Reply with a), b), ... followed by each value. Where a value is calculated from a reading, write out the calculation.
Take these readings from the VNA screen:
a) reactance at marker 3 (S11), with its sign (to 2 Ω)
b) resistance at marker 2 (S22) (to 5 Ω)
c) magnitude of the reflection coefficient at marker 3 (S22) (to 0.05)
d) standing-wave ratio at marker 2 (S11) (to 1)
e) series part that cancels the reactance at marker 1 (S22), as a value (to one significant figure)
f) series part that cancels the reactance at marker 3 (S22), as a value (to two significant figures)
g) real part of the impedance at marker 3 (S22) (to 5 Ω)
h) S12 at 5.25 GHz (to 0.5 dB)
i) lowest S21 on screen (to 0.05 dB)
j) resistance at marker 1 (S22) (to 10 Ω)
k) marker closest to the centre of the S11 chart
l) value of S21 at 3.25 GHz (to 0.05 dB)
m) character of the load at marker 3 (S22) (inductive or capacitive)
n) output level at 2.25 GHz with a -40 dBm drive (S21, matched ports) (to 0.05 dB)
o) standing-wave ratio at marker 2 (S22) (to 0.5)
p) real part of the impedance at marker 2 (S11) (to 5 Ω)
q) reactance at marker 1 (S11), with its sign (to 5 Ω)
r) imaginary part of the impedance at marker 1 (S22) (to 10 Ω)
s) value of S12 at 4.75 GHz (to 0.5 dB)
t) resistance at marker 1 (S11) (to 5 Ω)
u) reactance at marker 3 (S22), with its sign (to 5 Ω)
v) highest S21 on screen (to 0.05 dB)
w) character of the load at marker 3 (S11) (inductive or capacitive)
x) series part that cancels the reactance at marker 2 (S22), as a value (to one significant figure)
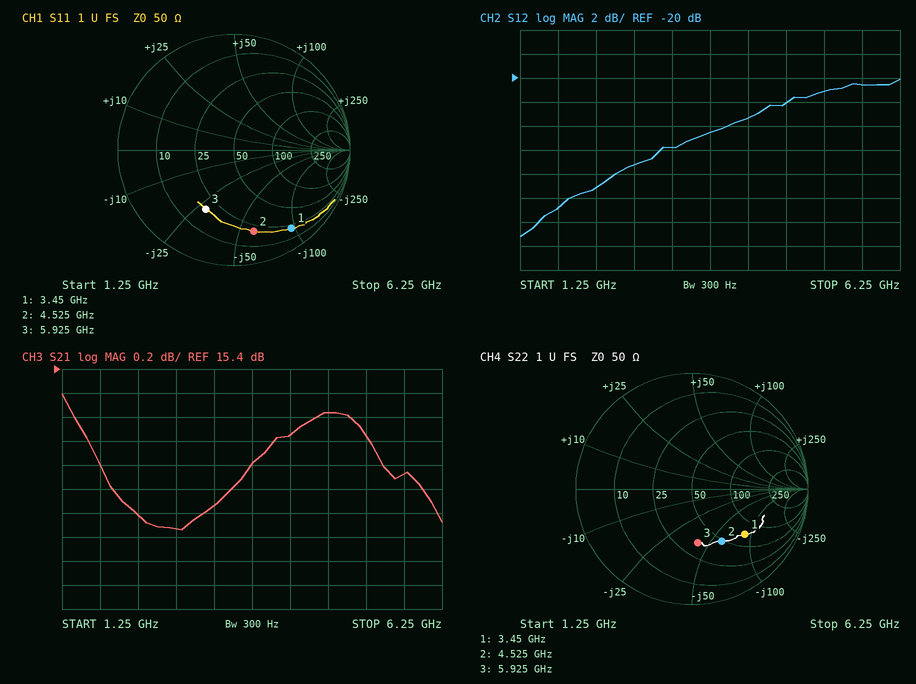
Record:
a) -28 Ω
b) 50 Ω
c) 0.45
d) 6
e) L = 90 Ω/(2π × 3.45 GHz) ≈ 4 nH
f) L = 40 Ω/(2π × 5.925 GHz) ≈ 1.1 nH
g) 35 Ω
h) -21.0 dB
i) 14.05 dB
j) 70 Ω
k) marker 3
l) 14.25 dB
m) capacitive
n) -40 dBm + (14.20 dB) = -25.80 dBm
o) 3.0
p) 20 Ω
q) -95 Ω
r) -90 Ω
s) -22.0 dB
t) 20 Ω
u) -40 Ω
v) 15.20 dB
w) capacitive
x) L = 60 Ω/(2π × 4.525 GHz) ≈ 2 nH
